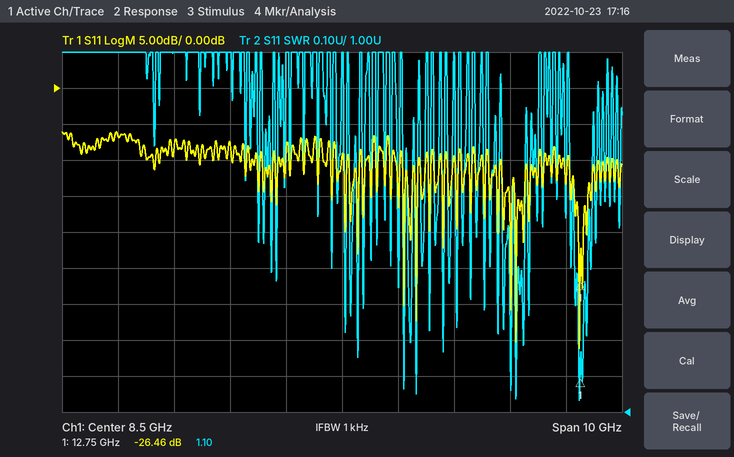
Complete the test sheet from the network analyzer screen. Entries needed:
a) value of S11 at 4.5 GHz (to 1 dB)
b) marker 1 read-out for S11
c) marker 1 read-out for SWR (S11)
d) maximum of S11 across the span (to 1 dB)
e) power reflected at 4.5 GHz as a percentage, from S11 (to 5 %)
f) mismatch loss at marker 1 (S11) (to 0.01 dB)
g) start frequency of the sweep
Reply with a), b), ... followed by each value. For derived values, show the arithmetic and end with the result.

a) -7 dB
b) -26.46 dB
c) 1.10
d) -6 dB
e) 10^(-7/10) ≈ 20 %
f) −10 log10(1 − 10^(-26.46/10)) ≈ 0.01 dB
g) 3.5 GHz
